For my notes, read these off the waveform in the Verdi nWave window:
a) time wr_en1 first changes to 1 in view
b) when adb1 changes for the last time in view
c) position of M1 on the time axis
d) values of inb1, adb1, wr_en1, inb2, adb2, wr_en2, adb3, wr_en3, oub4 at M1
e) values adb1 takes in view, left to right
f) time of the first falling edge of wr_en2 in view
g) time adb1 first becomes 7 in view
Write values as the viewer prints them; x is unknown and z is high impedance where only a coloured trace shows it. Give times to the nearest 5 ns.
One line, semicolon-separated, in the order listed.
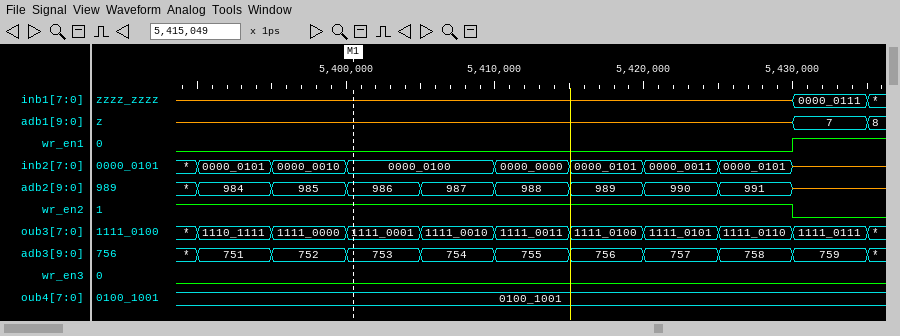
5430 ns; 5435 ns; 5400 ns; inb1=z, adb1=z, wr_en1=0, inb2=0000_0100, adb2=986, wr_en2=1, adb3=753, wr_en3=0, oub4=0100_1001; z, 7, 8; 5430 ns; 5430 ns
